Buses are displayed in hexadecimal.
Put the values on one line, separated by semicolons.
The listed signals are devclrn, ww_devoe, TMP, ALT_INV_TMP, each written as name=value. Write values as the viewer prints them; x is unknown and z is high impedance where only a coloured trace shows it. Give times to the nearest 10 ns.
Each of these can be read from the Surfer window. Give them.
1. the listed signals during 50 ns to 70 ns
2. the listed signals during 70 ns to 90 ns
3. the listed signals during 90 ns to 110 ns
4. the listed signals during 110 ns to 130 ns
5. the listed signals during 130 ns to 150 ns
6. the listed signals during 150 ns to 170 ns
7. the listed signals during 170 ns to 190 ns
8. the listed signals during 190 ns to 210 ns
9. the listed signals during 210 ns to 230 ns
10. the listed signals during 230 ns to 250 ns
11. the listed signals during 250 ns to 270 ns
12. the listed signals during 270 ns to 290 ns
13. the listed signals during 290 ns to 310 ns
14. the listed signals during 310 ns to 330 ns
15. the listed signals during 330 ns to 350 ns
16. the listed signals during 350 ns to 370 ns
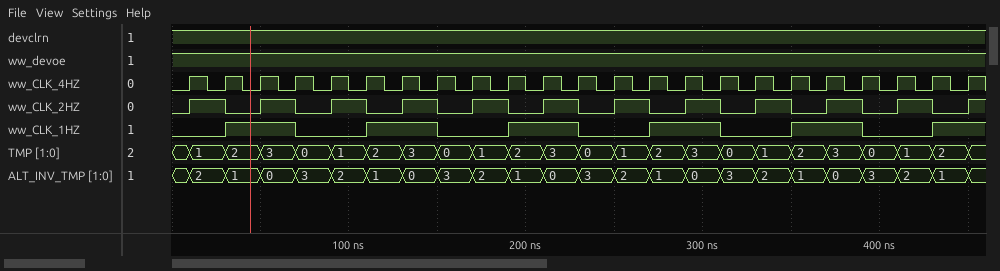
devclrn=1, ww_devoe=1, TMP=3, ALT_INV_TMP=0; devclrn=1, ww_devoe=1, TMP=0, ALT_INV_TMP=3; devclrn=1, ww_devoe=1, TMP=1, ALT_INV_TMP=2; devclrn=1, ww_devoe=1, TMP=2, ALT_INV_TMP=1; devclrn=1, ww_devoe=1, TMP=3, ALT_INV_TMP=0; devclrn=1, ww_devoe=1, TMP=0, ALT_INV_TMP=3; devclrn=1, ww_devoe=1, TMP=1, ALT_INV_TMP=2; devclrn=1, ww_devoe=1, TMP=2, ALT_INV_TMP=1; devclrn=1, ww_devoe=1, TMP=3, ALT_INV_TMP=0; devclrn=1, ww_devoe=1, TMP=0, ALT_INV_TMP=3; devclrn=1, ww_devoe=1, TMP=1, ALT_INV_TMP=2; devclrn=1, ww_devoe=1, TMP=2, ALT_INV_TMP=1; devclrn=1, ww_devoe=1, TMP=3, ALT_INV_TMP=0; devclrn=1, ww_devoe=1, TMP=0, ALT_INV_TMP=3; devclrn=1, ww_devoe=1, TMP=1, ALT_INV_TMP=2; devclrn=1, ww_devoe=1, TMP=2, ALT_INV_TMP=1
